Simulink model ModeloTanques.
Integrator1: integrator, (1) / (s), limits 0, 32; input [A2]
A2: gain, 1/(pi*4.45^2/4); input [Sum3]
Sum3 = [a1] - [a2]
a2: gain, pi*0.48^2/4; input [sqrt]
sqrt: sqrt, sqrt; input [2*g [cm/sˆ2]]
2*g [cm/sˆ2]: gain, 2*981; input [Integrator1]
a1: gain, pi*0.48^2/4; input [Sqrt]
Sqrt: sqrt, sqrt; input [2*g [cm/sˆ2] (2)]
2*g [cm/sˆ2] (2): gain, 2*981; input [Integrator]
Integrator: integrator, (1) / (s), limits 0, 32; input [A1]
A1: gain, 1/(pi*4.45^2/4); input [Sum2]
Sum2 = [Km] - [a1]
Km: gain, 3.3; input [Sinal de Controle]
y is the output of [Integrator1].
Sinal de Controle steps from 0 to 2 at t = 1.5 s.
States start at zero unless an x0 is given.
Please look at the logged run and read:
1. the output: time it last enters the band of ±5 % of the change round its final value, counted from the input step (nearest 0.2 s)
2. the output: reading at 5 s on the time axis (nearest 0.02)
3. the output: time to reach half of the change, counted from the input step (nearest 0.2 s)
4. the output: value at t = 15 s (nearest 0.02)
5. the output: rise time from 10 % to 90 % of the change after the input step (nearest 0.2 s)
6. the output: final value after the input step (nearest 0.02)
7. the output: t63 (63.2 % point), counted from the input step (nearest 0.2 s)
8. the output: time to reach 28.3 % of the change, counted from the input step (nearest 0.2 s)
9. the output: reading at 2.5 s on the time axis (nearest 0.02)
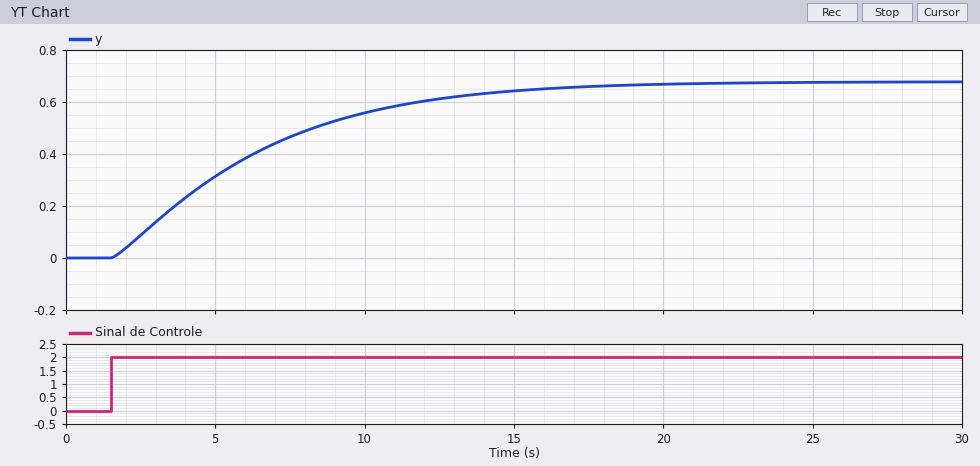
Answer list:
13.6 s
0.32
3.8 s
0.64
10.0 s
0.68
5.2 s
2.0 s
0.08
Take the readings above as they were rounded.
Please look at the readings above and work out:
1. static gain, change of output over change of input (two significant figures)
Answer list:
0.34
